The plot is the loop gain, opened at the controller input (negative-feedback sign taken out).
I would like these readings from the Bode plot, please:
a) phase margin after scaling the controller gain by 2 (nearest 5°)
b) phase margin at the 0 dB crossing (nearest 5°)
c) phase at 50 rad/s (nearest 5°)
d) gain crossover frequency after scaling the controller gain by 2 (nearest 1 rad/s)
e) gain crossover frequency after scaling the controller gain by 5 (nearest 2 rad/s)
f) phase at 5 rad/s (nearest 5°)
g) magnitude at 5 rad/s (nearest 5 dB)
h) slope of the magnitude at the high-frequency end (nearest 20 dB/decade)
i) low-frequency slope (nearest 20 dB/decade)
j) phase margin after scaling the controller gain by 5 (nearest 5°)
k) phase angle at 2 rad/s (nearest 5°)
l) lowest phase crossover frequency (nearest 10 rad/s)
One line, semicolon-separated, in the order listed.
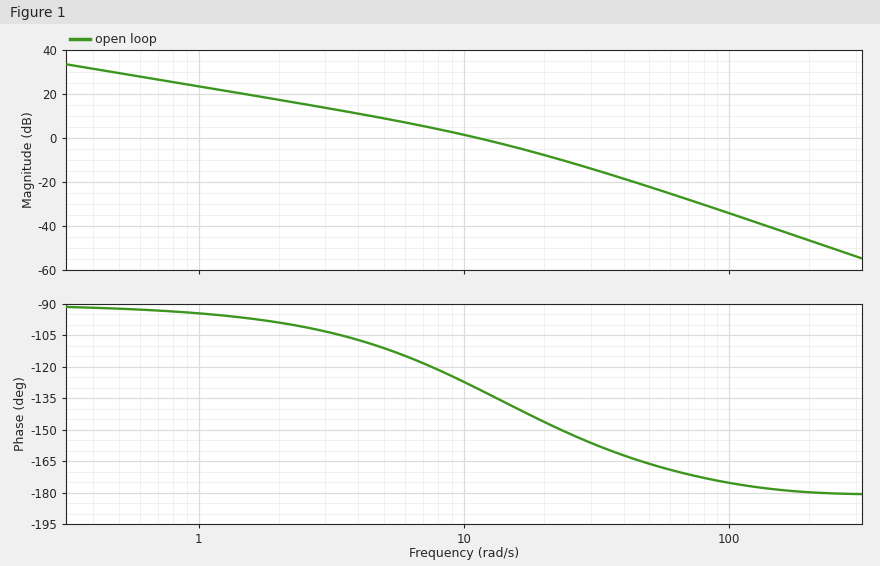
35°; 50°; -165°; 18 rad/s; 30 rad/s; -110°; 10 dB; -40 dB/decade; -20 dB/decade; 25°; -100°; 210 rad/s
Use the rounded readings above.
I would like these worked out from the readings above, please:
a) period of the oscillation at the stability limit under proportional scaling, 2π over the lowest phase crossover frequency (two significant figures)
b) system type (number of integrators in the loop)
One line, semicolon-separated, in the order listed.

0.030 s; 1
